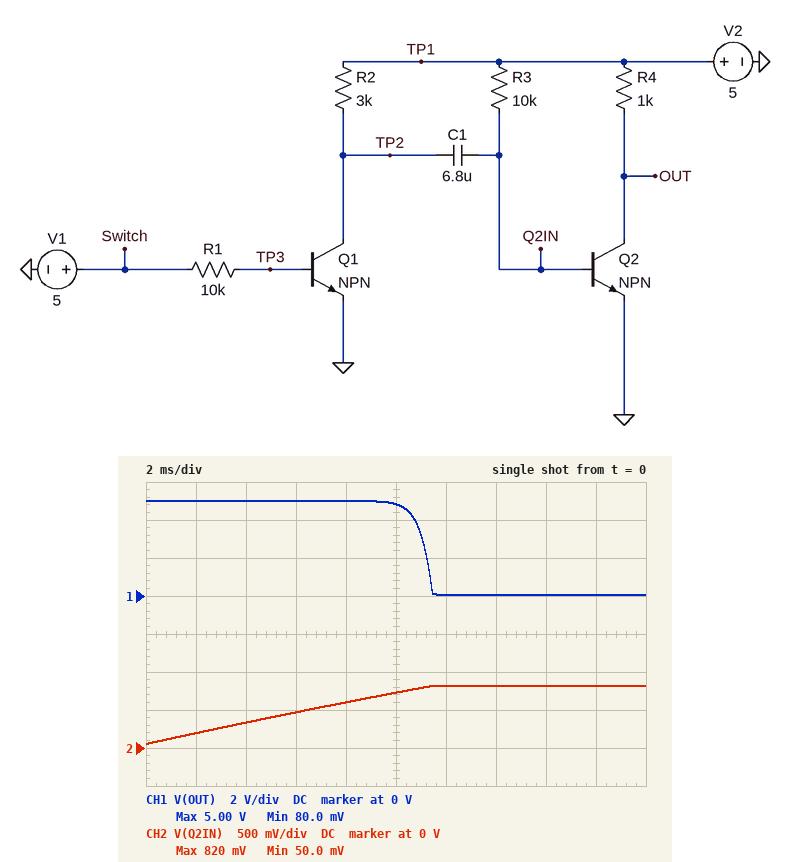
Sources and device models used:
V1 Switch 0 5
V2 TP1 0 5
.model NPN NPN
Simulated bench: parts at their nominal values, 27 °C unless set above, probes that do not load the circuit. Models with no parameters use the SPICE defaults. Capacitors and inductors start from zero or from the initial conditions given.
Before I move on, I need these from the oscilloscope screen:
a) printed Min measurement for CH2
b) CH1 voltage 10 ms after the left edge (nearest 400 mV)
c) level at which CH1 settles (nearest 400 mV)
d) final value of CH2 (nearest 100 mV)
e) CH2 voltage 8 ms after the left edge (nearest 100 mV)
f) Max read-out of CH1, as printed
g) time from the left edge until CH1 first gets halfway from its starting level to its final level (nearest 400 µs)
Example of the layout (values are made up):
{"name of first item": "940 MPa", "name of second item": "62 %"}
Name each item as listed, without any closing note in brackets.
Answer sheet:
{"printed Min measurement for CH2": "50.0 mV", "CH1 voltage 10 ms after the left edge": "4.8 V", "level at which CH1 settles": "0 V", "final value of CH2": "800 mV", "CH2 voltage 8 ms after the left edge": "600 mV", "Max read-out of CH1, as printed": "5.00 V", "time from the left edge until CH1 first gets halfway from its starting level to its final level": "11.2 ms"}
